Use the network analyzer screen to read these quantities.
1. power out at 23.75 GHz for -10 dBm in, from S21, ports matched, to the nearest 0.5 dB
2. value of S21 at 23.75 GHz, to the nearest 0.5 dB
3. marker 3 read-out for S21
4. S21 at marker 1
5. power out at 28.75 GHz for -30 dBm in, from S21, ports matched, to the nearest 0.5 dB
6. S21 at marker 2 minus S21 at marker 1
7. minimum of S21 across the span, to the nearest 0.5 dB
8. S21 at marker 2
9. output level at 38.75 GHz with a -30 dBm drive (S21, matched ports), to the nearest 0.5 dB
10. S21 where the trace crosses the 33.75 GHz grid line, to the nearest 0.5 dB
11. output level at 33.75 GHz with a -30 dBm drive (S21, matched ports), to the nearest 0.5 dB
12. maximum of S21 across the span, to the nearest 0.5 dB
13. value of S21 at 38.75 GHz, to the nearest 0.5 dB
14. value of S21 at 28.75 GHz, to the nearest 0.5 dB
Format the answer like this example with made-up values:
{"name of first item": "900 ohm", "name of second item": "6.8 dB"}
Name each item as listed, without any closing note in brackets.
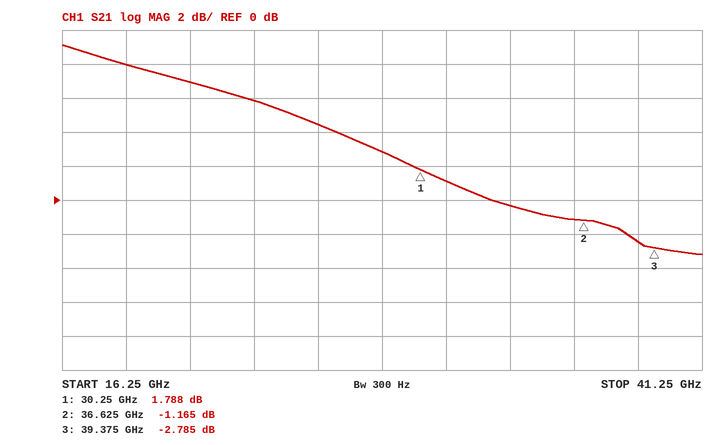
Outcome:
{"power out at 23.75 GHz for -10 dBm in, from S21, ports matched, to the nearest 0.5 dB": "-4.0 dBm", "value of S21 at 23.75 GHz, to the nearest 0.5 dB": "6.0 dB", "marker 3 read-out for S21": "-2.785 dB", "S21 at marker 1": "1.788 dB", "power out at 28.75 GHz for -30 dBm in, from S21, ports matched, to the nearest 0.5 dB": "-27.0 dBm", "S21 at marker 2 minus S21 at marker 1": "-2.953 dB", "minimum of S21 across the span, to the nearest 0.5 dB": "-3.0 dB", "S21 at marker 2": "-1.165 dB", "output level at 38.75 GHz with a -30 dBm drive (S21, matched ports), to the nearest 0.5 dB": "-32.5 dBm", "S21 where the trace crosses the 33.75 GHz grid line, to the nearest 0.5 dB": "-0.5 dB", "output level at 33.75 GHz with a -30 dBm drive (S21, matched ports), to the nearest 0.5 dB": "-30.5 dBm", "maximum of S21 across the span, to the nearest 0.5 dB": "9.0 dB", "value of S21 at 38.75 GHz, to the nearest 0.5 dB": "-2.5 dB", "value of S21 at 28.75 GHz, to the nearest 0.5 dB": "3.0 dB"}
